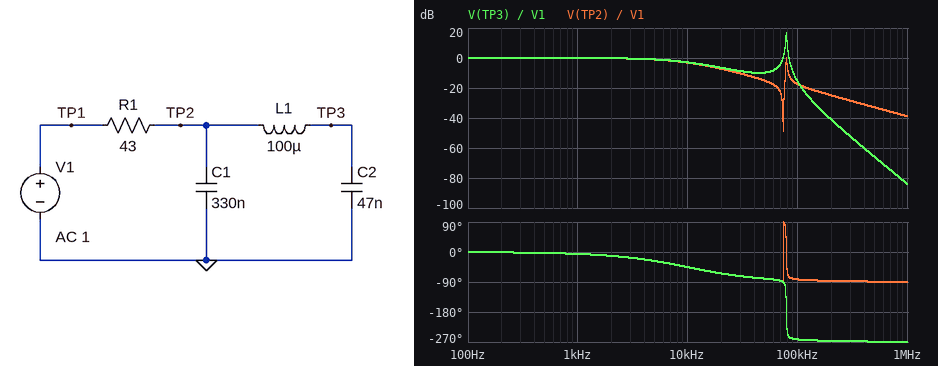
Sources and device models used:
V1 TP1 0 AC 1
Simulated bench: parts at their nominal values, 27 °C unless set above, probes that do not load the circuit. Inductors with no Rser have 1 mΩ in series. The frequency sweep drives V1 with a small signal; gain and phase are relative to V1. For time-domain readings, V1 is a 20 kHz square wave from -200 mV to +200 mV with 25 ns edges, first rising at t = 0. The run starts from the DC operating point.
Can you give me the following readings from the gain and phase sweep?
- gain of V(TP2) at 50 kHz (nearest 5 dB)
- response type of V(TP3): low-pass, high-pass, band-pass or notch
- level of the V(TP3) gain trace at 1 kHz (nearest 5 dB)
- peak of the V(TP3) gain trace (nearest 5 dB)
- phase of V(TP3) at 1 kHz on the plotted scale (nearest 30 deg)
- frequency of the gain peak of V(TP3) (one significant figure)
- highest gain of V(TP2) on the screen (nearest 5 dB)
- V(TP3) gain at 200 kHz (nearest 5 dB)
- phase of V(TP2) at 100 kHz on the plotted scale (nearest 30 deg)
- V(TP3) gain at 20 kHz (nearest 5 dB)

-15 dB
band-pass
0 dB
15 dB
0 deg
80 kHz
0 dB
-40 dB
-90 deg
-5 dB
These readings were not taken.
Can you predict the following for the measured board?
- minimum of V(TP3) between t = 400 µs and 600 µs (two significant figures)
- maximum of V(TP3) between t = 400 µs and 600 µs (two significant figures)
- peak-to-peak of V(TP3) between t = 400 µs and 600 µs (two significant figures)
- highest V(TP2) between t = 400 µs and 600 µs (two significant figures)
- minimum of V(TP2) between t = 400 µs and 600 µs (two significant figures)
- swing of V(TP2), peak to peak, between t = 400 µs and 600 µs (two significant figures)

-140 mV
140 mV
290 mV
130 mV
-130 mV
260 mV
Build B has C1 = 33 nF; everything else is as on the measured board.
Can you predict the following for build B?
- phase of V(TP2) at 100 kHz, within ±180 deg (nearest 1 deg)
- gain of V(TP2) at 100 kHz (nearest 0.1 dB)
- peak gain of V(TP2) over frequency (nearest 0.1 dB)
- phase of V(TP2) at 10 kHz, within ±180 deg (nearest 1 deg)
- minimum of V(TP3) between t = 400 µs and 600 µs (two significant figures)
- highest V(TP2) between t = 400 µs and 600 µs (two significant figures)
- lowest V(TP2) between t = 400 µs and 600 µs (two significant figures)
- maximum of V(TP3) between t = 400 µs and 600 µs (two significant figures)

31 deg
-1.3 dB
0 dB
-12 deg
-250 mV
240 mV
-240 mV
250 mV
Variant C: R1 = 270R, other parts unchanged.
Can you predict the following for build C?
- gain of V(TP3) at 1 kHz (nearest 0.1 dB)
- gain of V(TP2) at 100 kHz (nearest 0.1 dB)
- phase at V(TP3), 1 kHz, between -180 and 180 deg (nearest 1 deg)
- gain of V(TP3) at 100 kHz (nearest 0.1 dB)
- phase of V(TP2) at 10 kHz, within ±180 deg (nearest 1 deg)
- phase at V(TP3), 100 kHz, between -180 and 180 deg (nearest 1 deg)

-1.5 dB
-33.4 dB
-33 deg
-32.0 dB
-81 deg
91 deg
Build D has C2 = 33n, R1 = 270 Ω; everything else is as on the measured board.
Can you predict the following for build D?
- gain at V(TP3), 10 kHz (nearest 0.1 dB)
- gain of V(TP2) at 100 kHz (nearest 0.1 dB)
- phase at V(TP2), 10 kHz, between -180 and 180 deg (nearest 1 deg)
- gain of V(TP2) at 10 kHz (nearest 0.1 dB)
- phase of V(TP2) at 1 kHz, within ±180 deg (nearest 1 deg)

-15.8 dB
-31.5 dB
-81 deg
-15.9 dB
-32 deg
